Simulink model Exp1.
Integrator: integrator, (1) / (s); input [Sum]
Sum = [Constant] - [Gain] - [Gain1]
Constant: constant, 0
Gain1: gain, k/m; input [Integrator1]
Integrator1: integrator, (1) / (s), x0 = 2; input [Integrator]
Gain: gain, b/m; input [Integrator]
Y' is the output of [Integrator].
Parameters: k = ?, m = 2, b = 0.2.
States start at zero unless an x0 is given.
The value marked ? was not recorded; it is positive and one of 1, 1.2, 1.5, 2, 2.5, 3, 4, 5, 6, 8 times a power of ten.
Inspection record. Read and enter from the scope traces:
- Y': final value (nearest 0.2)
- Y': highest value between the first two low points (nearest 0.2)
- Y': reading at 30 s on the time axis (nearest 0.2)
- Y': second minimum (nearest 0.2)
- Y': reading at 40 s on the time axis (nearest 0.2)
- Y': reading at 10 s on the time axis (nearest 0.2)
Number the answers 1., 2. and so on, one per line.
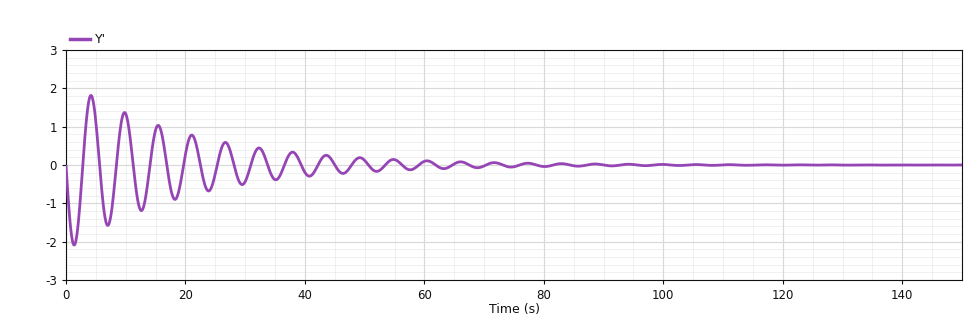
1. 0.0
2. 1.8
3. -0.4
4. -1.6
5. -0.2
6. 1.4
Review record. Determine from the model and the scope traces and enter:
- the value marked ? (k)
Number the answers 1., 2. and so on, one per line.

1. 2.5
